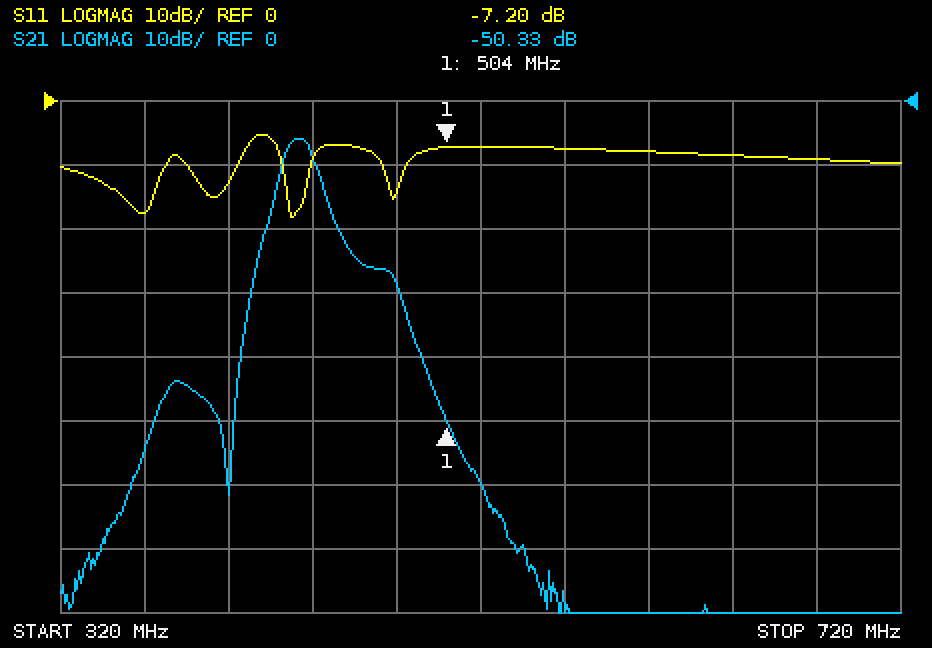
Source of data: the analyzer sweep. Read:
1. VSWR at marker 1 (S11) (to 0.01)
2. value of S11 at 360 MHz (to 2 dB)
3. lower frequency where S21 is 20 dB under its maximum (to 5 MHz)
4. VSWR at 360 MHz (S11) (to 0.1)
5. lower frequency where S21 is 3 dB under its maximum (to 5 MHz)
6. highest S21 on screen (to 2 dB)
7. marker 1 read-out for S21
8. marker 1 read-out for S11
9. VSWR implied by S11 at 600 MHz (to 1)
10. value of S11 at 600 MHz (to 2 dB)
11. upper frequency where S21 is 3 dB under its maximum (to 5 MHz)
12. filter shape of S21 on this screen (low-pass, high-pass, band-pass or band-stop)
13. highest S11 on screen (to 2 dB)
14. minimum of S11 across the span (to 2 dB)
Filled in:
2.55
-18 dB
415 MHz
1.3
425 MHz
-6 dB
-50.33 dB
-7.20 dB
2
-8 dB
440 MHz
band-pass
-6 dB
-18 dB
